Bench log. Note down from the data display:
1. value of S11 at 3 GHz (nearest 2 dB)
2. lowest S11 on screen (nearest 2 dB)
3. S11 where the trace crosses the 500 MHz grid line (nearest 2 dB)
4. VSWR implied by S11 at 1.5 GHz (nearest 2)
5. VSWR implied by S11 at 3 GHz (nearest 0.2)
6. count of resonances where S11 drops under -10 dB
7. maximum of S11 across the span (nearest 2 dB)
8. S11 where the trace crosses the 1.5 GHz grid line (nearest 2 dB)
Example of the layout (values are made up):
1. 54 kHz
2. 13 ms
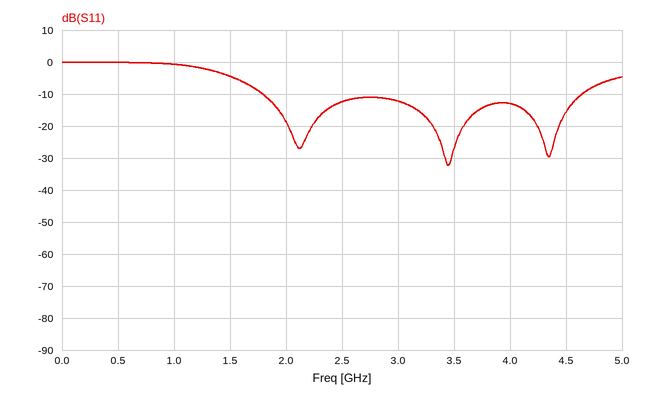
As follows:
1. -12 dB
2. -32 dB
3. 0 dB
4. 4
5. 1.6
6. 3
7. 0 dB
8. -4 dB
